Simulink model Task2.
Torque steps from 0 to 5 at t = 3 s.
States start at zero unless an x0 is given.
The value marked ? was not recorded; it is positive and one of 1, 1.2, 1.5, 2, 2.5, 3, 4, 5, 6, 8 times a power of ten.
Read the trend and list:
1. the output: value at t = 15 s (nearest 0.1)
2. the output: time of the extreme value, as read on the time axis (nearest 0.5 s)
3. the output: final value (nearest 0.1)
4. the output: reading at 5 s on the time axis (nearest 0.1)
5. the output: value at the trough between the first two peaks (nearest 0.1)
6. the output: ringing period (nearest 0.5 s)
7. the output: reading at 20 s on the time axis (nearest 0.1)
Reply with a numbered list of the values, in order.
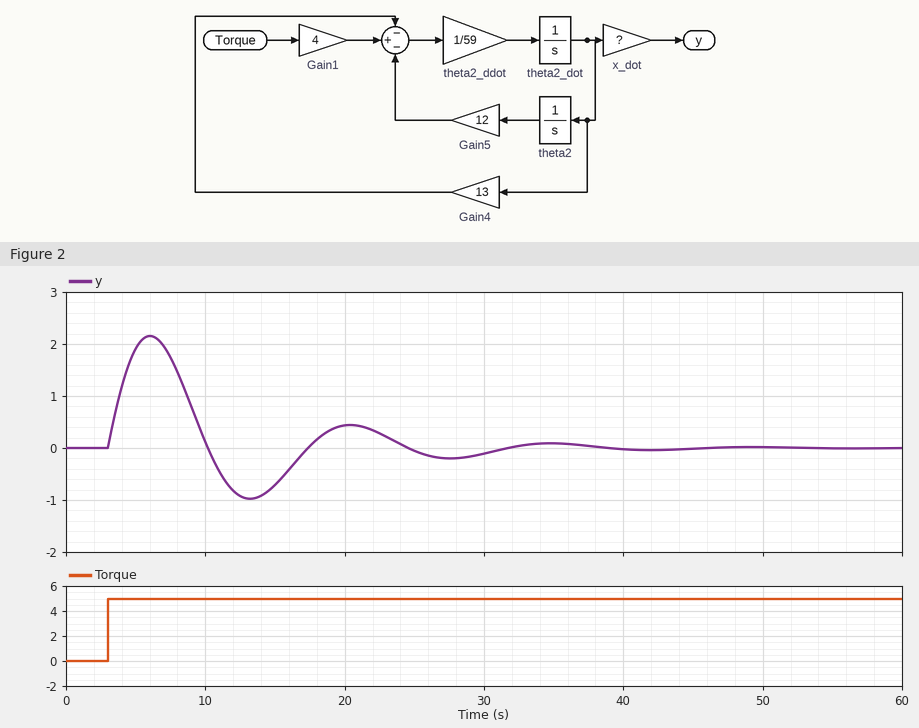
1. -0.7
2. 6.0 s
3. 0.0
4. 1.9
5. -1.0
6. 14.5 s
7. 0.4
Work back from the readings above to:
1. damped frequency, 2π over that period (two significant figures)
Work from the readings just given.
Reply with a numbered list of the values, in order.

1. 0.43 rad/s
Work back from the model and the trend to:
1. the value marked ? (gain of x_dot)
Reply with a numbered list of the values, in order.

1. 4
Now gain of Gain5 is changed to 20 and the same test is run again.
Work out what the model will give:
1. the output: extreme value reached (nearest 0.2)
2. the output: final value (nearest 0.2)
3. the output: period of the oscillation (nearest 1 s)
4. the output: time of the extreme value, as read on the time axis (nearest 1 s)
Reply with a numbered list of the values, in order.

1. 1.8
2. 0.0
3. 11 s
4. 5 s
